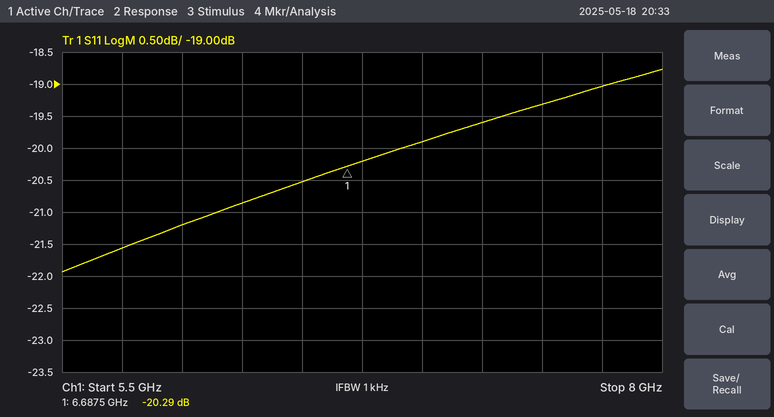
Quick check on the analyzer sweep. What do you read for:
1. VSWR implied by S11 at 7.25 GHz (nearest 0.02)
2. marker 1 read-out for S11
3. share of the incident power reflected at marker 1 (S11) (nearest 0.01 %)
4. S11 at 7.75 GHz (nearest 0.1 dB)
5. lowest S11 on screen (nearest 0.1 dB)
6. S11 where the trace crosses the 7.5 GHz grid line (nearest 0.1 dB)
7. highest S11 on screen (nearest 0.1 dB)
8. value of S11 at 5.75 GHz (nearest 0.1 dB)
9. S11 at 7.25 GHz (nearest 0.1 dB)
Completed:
1.24
-20.29 dB
0.94 %
-19.0 dB
-21.9 dB
-19.3 dB
-18.8 dB
-21.6 dB
-19.6 dB
